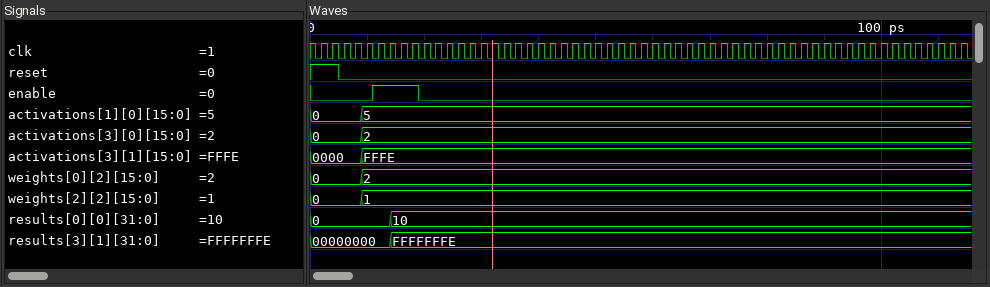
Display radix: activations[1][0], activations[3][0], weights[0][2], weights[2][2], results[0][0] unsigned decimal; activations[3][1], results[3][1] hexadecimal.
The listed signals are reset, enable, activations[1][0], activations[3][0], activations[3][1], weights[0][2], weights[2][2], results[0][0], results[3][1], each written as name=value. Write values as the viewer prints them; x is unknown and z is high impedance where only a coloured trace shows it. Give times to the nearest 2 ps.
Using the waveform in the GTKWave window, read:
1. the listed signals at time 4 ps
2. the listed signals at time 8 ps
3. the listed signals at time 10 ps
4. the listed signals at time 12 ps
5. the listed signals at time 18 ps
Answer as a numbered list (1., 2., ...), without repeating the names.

1. reset=1, enable=0, activations[1][0]=0, activations[3][0]=0, activations[3][1]=0000, weights[0][2]=0, weights[2][2]=0, results[0][0]=0, results[3][1]=00000000
2. reset=0, enable=0, activations[1][0]=0, activations[3][0]=0, activations[3][1]=0000, weights[0][2]=0, weights[2][2]=0, results[0][0]=0, results[3][1]=00000000
3. reset=0, enable=0, activations[1][0]=5, activations[3][0]=2, activations[3][1]=FFFE, weights[0][2]=2, weights[2][2]=1, results[0][0]=0, results[3][1]=00000000
4. reset=0, enable=1, activations[1][0]=5, activations[3][0]=2, activations[3][1]=FFFE, weights[0][2]=2, weights[2][2]=1, results[0][0]=0, results[3][1]=00000000
5. reset=0, enable=1, activations[1][0]=5, activations[3][0]=2, activations[3][1]=FFFE, weights[0][2]=2, weights[2][2]=1, results[0][0]=10, results[3][1]=FFFFFFFE
